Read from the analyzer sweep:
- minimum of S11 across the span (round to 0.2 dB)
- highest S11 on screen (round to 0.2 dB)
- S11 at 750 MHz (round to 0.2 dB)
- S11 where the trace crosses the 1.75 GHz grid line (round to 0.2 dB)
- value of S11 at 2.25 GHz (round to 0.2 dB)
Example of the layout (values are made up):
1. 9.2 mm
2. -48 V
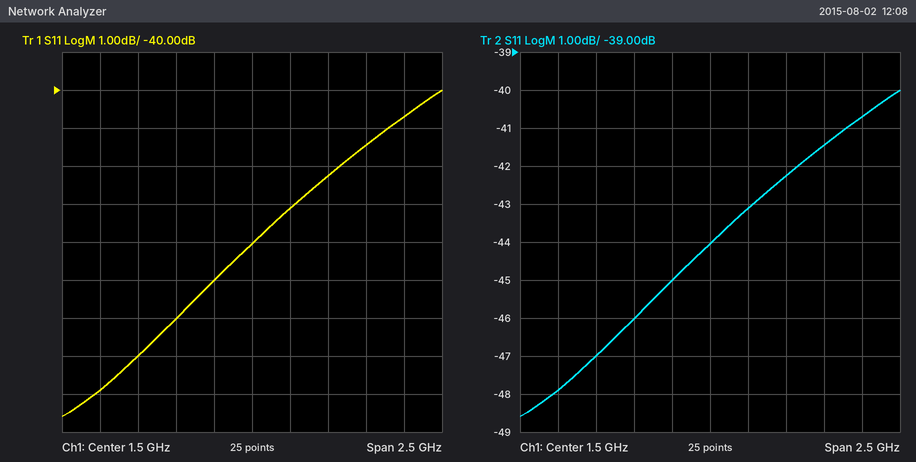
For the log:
1. -48.6 dB
2. -40.0 dB
3. -47.0 dB
4. -43.2 dB
5. -41.4 dB
